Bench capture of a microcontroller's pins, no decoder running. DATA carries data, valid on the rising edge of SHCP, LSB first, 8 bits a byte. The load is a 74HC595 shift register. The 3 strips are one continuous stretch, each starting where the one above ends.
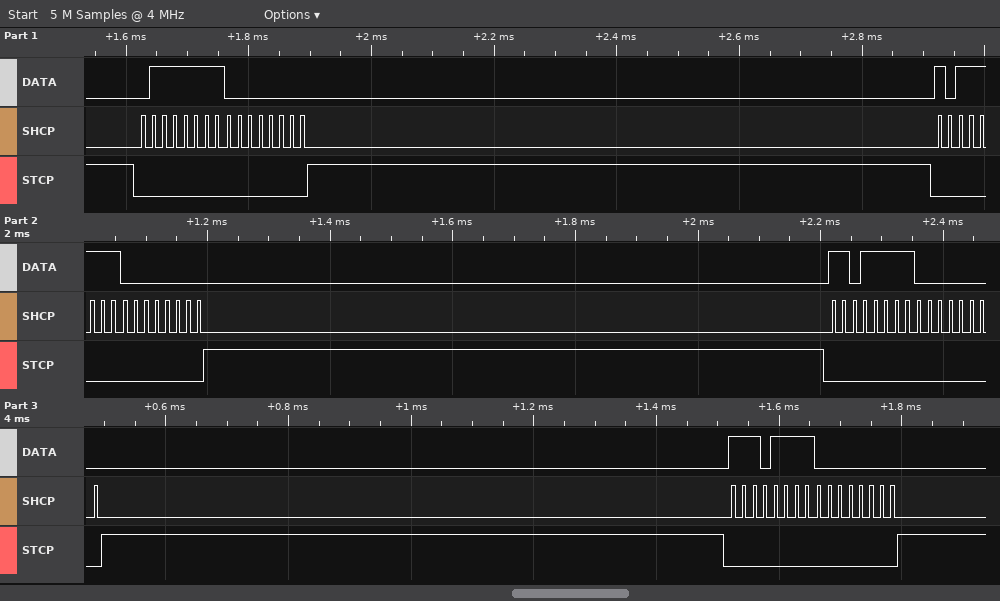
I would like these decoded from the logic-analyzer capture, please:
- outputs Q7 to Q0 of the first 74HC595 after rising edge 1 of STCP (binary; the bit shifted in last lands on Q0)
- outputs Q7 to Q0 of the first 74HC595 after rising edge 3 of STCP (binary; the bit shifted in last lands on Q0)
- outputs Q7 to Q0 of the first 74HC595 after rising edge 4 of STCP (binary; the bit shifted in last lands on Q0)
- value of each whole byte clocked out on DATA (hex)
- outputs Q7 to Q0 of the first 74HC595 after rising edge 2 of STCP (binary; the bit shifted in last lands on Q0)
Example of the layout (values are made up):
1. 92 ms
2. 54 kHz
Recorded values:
1. 00000000
2. 00000000
3. 00000000
4. FE 00 FD 00 FB 00 F7 00
5. 00000000
